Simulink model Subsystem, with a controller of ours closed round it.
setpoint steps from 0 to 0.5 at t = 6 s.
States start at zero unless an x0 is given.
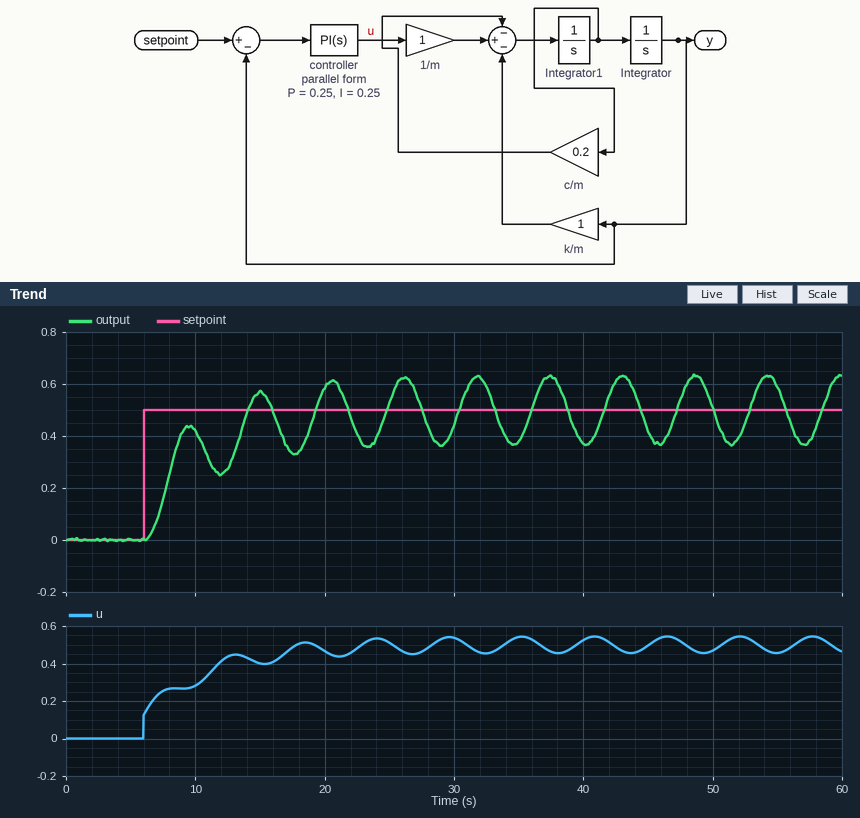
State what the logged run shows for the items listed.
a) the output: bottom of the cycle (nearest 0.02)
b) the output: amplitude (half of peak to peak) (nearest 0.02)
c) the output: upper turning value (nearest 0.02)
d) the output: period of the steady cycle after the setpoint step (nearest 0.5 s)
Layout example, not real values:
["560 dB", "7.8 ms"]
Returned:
["0.36", "0.14", "0.64", "5.5 s"]
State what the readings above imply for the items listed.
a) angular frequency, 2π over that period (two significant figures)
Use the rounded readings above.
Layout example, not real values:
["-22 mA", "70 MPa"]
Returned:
["1.1 rad/s"]
